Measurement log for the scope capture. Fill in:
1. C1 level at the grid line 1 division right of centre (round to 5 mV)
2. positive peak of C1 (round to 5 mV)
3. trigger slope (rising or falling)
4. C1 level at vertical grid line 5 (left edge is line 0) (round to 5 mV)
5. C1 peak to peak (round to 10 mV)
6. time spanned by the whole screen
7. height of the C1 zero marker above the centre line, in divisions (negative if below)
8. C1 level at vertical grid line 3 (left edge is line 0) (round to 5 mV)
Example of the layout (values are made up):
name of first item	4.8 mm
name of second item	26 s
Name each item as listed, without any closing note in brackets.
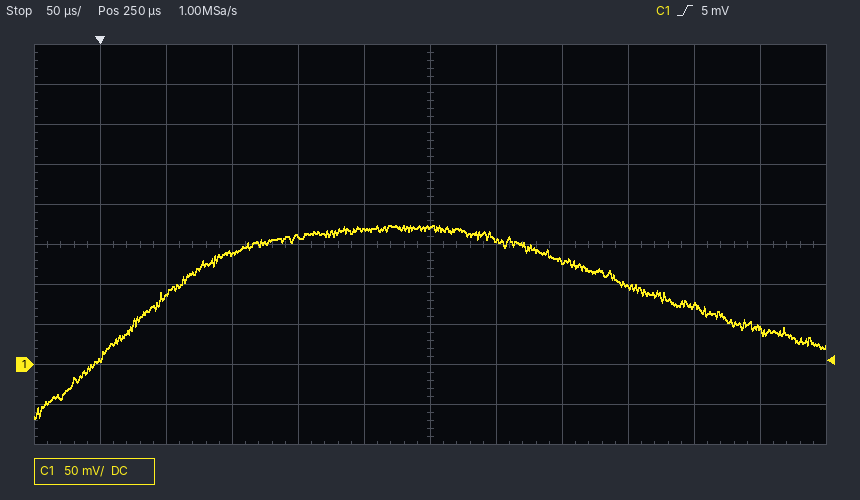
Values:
C1 level at the grid line 1 division right of centre	155 mV
positive peak of C1	175 mV
trigger slope	rising
C1 level at vertical grid line 5 (left edge is line 0)	170 mV
C1 peak to peak	240 mV
time spanned by the whole screen	600 µs
height of the C1 zero marker above the centre line, in divisions	-3.0 div
C1 level at vertical grid line 3 (left edge is line 0)	140 mV
